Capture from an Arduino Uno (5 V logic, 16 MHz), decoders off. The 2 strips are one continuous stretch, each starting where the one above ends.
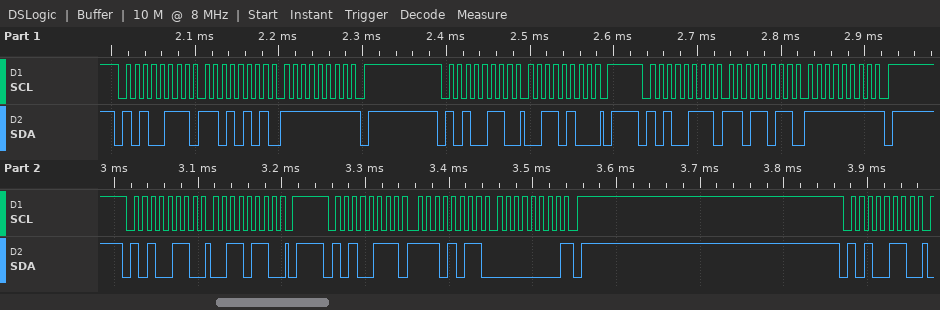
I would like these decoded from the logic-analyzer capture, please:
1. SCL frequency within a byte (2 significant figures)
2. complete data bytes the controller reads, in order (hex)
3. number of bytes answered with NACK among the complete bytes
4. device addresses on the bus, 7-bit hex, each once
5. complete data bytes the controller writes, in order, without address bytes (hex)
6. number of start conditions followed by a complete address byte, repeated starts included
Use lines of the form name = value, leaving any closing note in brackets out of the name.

SCL frequency within a byte = 100 kHz
complete data bytes the controller reads, in order = D5 FF DB FF EB 00
number of bytes answered with NACK among the complete bytes = 3
device addresses on the bus, 7-bit hex, each once = 0x53
complete data bytes the controller writes, in order, without address bytes = 34 36
number of start conditions followed by a complete address byte, repeated starts included = 6
